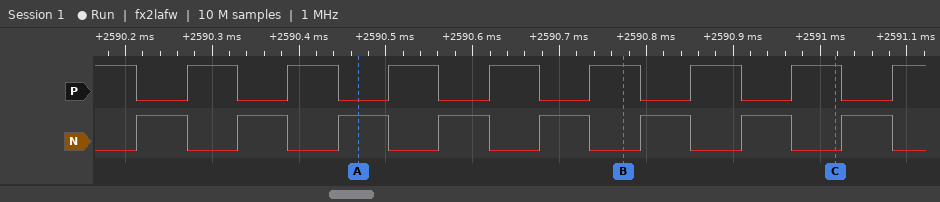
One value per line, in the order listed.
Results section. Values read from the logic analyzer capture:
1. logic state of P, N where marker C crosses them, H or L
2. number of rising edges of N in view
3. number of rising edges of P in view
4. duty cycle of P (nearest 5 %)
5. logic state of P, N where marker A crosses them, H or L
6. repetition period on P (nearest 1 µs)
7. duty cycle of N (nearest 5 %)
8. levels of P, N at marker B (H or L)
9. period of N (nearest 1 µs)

P=H, N=L
8
8
50 %
P=L, N=H
116 µs
50 %
P=H, N=L
116 µs
